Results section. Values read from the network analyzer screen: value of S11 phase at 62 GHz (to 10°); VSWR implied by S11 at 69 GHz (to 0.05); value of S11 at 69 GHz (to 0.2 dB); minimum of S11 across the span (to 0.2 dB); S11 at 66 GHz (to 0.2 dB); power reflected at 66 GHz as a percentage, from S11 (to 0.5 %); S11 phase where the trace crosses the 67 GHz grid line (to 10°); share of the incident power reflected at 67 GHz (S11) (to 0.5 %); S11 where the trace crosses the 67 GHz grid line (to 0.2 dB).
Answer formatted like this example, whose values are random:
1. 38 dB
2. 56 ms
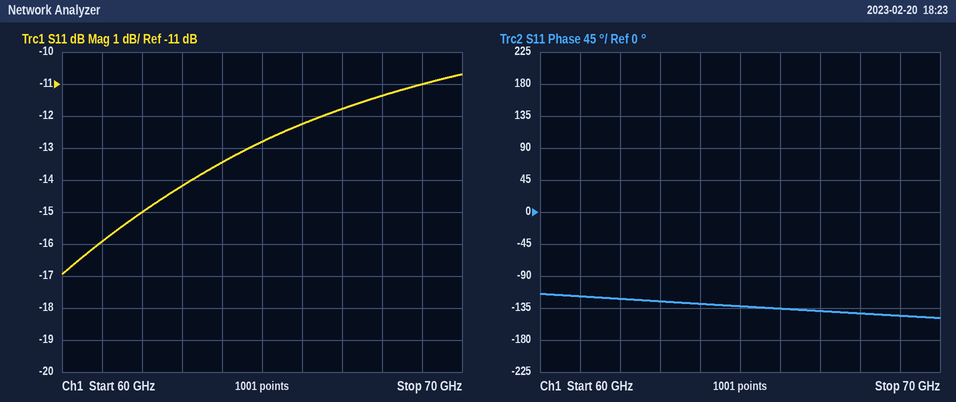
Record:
1. -120°
2. 1.80
3. -11.0 dB
4. -17.0 dB
5. -12.2 dB
6. 6.0 %
7. -140°
8. 6.5 %
9. -11.8 dB
